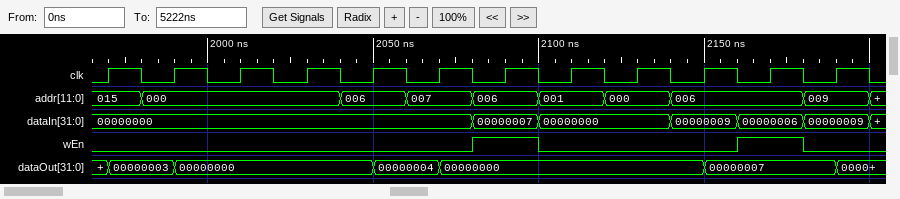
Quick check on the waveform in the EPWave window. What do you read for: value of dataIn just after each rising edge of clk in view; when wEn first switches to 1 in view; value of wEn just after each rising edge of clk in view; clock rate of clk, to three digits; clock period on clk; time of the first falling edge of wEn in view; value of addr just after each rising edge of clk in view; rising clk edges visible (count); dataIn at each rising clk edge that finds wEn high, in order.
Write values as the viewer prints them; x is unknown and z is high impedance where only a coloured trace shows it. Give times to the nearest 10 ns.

00000000, 00000000, 00000000, 00000000, 00000000, 00000000, 00000007, 00000000, 00000000, 00000009, 00000006, 00000009
2080 ns
0 0 0 0 0 0 1 0 0 0 1 0
50.0 MHz
20 ns
2100 ns
015, 000, 000, 000, 006, 007, 006, 001, 000, 006, 006, 009
12
00000007, 00000006
